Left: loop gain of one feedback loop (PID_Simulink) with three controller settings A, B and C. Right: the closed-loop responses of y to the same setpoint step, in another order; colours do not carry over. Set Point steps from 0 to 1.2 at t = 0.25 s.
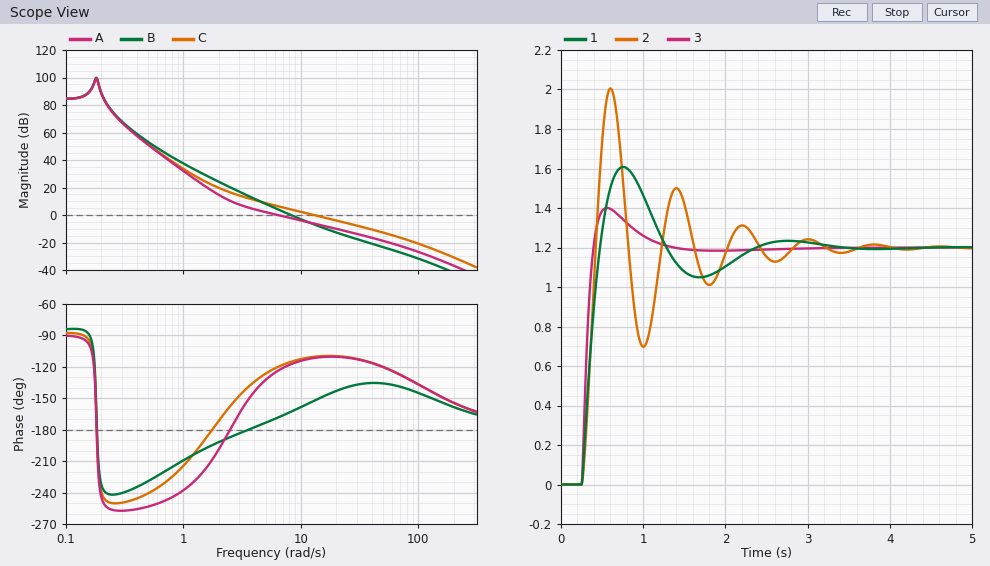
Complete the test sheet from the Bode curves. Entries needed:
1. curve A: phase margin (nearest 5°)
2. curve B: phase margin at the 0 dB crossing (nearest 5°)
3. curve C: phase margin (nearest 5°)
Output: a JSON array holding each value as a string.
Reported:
["55°", "15°", "70°"]
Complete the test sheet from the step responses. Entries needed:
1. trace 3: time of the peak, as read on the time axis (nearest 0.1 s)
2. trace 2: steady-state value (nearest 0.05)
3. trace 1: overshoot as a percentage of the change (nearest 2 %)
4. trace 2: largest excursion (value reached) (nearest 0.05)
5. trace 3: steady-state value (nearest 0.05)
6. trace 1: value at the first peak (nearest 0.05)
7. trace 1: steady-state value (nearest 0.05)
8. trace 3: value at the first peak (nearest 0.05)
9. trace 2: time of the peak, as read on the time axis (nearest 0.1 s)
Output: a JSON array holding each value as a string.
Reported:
["0.6 s", "1.20", "34 %", "2.00", "1.20", "1.60", "1.20", "1.40", "0.6 s"]
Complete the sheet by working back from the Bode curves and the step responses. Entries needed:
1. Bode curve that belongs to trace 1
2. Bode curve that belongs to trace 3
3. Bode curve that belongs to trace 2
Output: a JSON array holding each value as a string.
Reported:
["A", "C", "B"]
